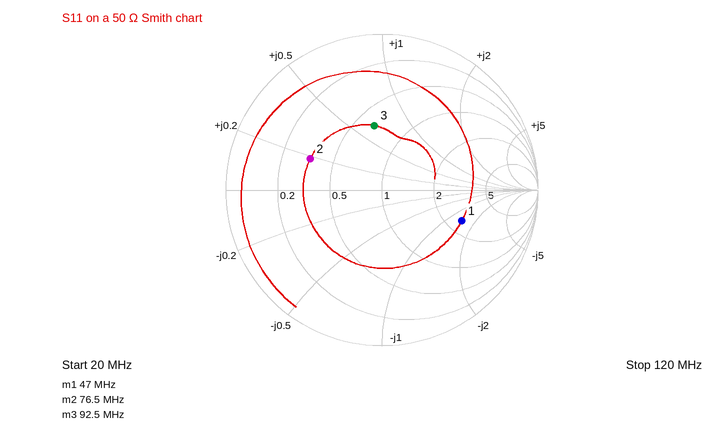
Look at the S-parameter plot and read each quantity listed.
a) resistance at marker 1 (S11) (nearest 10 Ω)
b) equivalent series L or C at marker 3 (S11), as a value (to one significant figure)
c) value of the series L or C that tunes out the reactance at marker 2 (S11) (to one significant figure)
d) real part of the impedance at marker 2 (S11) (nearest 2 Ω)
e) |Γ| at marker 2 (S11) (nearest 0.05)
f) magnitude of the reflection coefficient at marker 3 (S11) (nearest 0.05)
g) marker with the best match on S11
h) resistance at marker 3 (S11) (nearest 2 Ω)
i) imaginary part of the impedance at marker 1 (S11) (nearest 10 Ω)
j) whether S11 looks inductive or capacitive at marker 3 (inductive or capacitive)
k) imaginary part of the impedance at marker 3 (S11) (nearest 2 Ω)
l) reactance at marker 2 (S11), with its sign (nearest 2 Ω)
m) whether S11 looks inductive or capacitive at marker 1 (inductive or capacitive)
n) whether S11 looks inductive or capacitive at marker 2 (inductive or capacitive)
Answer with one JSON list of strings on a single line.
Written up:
["130 Ω", "60 nH", "200 pF", "18 Ω", "0.50", "0.40", "marker 3", "32 Ω", "-70 Ω", "inductive", "+32 Ω", "+10 Ω", "capacitive", "inductive"]
